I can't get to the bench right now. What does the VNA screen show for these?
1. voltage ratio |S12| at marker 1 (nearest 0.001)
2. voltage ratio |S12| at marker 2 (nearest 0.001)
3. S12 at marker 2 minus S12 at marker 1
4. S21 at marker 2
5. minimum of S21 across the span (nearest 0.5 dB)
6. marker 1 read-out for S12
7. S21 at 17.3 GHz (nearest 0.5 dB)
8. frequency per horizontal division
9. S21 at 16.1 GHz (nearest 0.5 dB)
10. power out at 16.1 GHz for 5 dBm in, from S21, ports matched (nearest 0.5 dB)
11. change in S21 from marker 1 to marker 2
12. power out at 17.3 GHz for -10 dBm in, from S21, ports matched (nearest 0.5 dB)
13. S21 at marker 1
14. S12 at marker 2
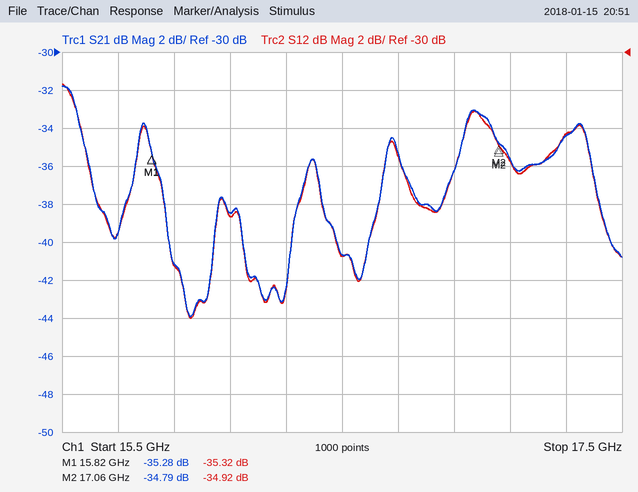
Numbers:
0.017
0.018
0.40 dB
-34.79 dB
-44.0 dB
-35.32 dB
-34.5 dB
200 MHz
-38.5 dB
-33.5 dBm
0.49 dB
-44.5 dBm
-35.28 dB
-34.92 dB
